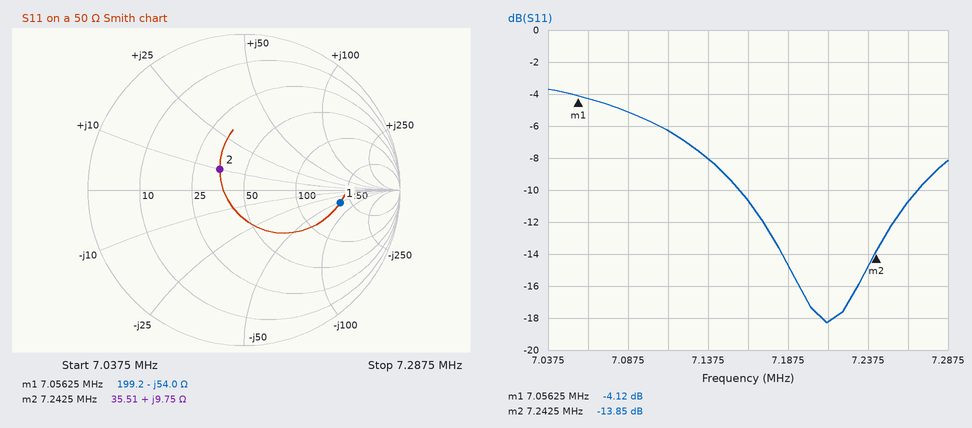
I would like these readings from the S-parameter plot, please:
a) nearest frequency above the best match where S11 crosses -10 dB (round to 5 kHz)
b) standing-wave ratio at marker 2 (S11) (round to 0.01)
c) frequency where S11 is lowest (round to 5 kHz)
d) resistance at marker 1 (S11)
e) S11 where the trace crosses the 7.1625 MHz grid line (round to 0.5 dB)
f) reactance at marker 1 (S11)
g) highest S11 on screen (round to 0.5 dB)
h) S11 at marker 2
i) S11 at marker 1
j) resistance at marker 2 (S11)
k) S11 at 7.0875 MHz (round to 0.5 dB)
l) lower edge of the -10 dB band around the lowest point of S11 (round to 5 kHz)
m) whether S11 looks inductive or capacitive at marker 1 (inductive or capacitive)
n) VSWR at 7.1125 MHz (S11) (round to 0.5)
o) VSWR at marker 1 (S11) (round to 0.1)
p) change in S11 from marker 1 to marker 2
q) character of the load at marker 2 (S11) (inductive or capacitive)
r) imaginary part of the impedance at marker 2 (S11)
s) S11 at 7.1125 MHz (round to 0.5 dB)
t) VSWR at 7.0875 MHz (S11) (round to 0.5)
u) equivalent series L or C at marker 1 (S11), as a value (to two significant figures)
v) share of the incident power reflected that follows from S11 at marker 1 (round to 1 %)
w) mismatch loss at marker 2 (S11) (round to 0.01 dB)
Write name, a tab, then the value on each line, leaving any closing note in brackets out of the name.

nearest frequency above the best match where S11 crosses -10 dB	7.270 MHz
standing-wave ratio at marker 2 (S11)	1.51
frequency where S11 is lowest	7.210 MHz
resistance at marker 1	199.2 Ω
S11 where the trace crosses the 7.1625 MHz grid line	-10.5 dB
reactance at marker 1	-54.0 Ω
highest S11 on screen	-3.5 dB
S11 at marker 2	-13.85 dB
S11 at marker 1	-4.12 dB
resistance at marker 2	35.51 Ω
S11 at 7.0875 MHz	-5.0 dB
lower edge of the -10 dB band around the lowest point of S11	7.155 MHz
whether S11 looks inductive or capacitive at marker 1	capacitive
VSWR at 7.1125 MHz (S11)	3.0
VSWR at marker 1 (S11)	4.3
change in S11 from marker 1 to marker 2	-9.73 dB
character of the load at marker 2 (S11)	inductive
imaginary part of the impedance at marker 2	+9.75 Ω
S11 at 7.1125 MHz	-6.5 dB
VSWR at 7.0875 MHz (S11)	3.5
equivalent series L or C at marker 1 (S11), as a value	420 pF
share of the incident power reflected that follows from S11 at marker 1	39 %
mismatch loss at marker 2 (S11)	0.18 dB
